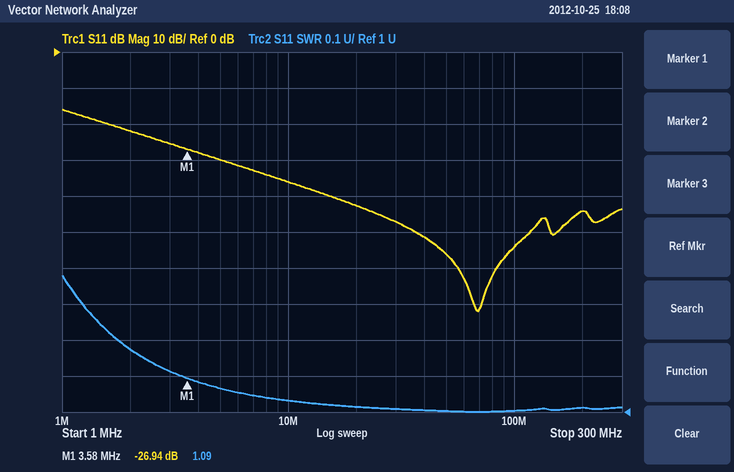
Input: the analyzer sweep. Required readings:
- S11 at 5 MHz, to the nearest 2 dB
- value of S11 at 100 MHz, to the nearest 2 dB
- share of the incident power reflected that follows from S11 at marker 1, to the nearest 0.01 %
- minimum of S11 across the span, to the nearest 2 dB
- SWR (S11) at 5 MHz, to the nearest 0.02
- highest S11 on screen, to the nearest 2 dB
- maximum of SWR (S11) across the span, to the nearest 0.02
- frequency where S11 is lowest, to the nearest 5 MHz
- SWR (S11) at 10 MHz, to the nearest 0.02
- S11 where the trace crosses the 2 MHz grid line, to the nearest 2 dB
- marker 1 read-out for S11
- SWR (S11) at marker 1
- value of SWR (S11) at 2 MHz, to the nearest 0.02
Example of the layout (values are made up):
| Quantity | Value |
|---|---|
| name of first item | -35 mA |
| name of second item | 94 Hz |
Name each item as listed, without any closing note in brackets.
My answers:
| Quantity | Value |
|---|---|
| S11 at 5 MHz, to the nearest 2 dB | -30 dB |
| value of S11 at 100 MHz, to the nearest 2 dB | -54 dB |
| share of the incident power reflected that follows from S11 at marker 1, to the nearest 0.01 % | 0.20 % |
| minimum of S11 across the span, to the nearest 2 dB | -72 dB |
| SWR (S11) at 5 MHz, to the nearest 0.02 | 1.06 |
| highest S11 on screen, to the nearest 2 dB | -16 dB |
| maximum of SWR (S11) across the span, to the nearest 0.02 | 1.38 |
| frequency where S11 is lowest, to the nearest 5 MHz | 70 MHz |
| SWR (S11) at 10 MHz, to the nearest 0.02 | 1.04 |
| S11 where the trace crosses the 2 MHz grid line, to the nearest 2 dB | -22 dB |
| marker 1 read-out for S11 | -26.94 dB |
| SWR (S11) at marker 1 | 1.09 |
| value of SWR (S11) at 2 MHz, to the nearest 0.02 | 1.18 |
